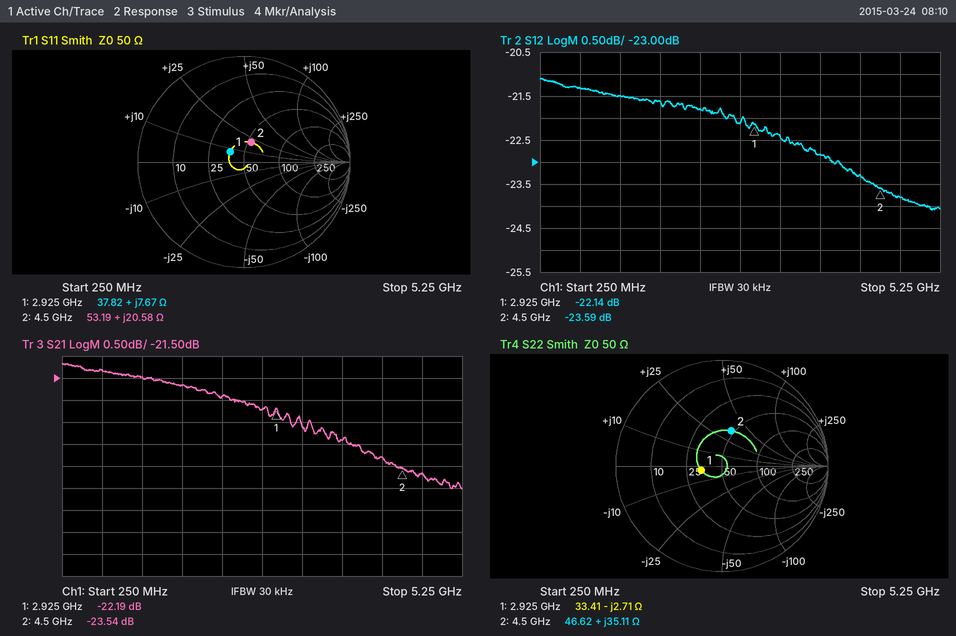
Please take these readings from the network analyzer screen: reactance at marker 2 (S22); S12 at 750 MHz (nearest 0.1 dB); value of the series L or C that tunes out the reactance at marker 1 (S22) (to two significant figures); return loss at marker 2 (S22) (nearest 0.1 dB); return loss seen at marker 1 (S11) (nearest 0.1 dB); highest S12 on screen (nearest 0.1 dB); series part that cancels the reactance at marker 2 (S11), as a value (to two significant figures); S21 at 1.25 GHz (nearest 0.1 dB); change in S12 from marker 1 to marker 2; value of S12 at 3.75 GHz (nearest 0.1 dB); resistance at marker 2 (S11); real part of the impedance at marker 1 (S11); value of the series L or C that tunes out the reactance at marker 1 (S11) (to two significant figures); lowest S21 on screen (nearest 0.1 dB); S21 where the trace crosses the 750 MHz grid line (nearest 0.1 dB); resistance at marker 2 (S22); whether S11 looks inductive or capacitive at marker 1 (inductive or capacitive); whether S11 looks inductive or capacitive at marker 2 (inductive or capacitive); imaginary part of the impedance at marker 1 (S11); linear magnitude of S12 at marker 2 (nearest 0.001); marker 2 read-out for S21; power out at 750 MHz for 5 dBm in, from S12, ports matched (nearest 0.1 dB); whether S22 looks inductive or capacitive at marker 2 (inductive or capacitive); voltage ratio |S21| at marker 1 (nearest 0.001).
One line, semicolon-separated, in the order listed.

+35.11 Ω; -21.3 dB; 150 pH; 9.3 dB; 15.7 dB; -21.1 dB; 1.7 pF; -21.5 dB; -1.45 dB; -22.8 dB; 53.19 Ω; 37.82 Ω; 7.1 pF; -24.0 dB; -21.3 dB; 46.62 Ω; inductive; inductive; +7.67 Ω; 0.066; -23.54 dB; -16.3 dBm; inductive; 0.078
